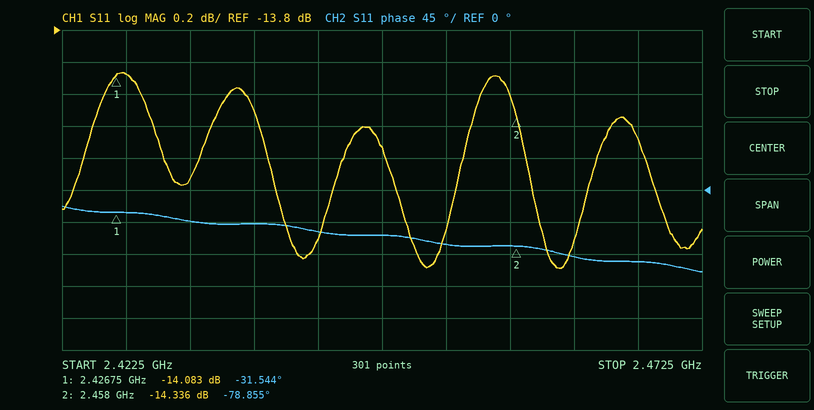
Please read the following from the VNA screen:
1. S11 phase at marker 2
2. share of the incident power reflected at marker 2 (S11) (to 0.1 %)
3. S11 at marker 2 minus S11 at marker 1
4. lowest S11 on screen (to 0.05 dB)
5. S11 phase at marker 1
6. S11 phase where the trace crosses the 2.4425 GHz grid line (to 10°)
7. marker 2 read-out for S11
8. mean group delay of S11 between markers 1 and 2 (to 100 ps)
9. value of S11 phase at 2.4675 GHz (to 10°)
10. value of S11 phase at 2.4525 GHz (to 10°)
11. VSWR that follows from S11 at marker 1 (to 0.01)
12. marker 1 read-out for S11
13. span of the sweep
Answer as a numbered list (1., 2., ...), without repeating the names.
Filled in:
1. -78.855°
2. 3.7 %
3. -0.253 dB
4. -15.30 dB
5. -31.544°
6. -60°
7. -14.336 dB
8. 4.2 ns
9. -100°
10. -80°
11. 1.49
12. -14.083 dB
13. 50 MHz
